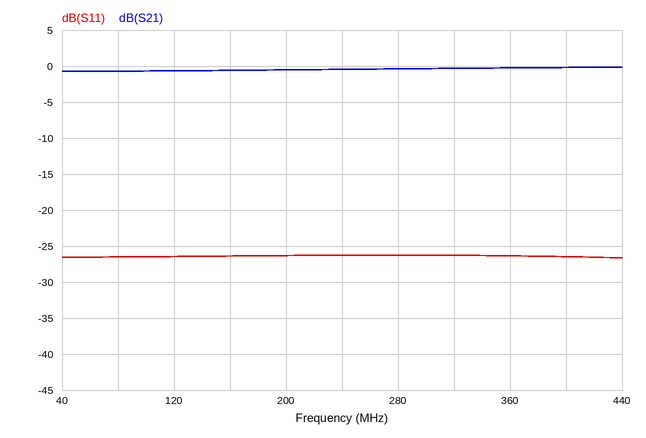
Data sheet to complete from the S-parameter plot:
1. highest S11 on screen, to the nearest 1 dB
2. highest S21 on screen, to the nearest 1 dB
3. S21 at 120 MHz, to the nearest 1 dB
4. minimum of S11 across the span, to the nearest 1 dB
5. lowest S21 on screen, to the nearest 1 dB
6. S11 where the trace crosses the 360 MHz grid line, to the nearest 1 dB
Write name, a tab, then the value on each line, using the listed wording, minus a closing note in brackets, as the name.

highest S11 on screen, to the nearest 1 dB	-26 dB
highest S21 on screen, to the nearest 1 dB	0 dB
S21 at 120 MHz, to the nearest 1 dB	-1 dB
minimum of S11 across the span, to the nearest 1 dB	-27 dB
lowest S21 on screen, to the nearest 1 dB	-1 dB
S11 where the trace crosses the 360 MHz grid line, to the nearest 1 dB	-26 dB
